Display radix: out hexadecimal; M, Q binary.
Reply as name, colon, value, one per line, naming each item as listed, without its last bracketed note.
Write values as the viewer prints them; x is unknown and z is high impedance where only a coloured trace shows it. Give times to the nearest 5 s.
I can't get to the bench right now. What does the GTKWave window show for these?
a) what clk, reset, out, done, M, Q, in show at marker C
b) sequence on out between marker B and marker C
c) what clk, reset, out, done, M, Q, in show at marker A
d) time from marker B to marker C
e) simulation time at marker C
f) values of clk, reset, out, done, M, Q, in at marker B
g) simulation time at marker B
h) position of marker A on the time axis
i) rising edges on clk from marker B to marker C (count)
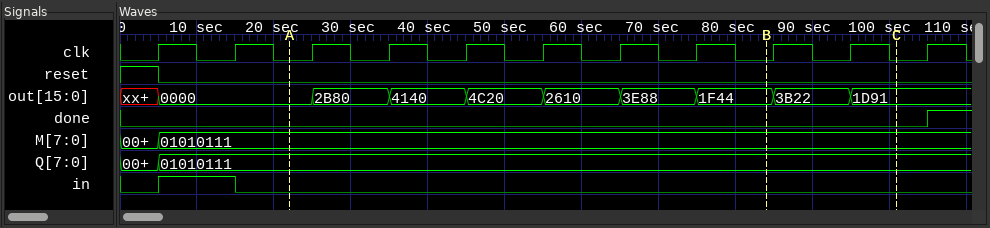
what clk, reset, out, done, M, Q, in show at marker C: clk=0, reset=0, out=1D91, done=0, M=01010111, Q=01010111, in=0
sequence on out between marker B and marker C: 1F44, 3B22, 1D91
what clk, reset, out, done, M, Q, in show at marker A: clk=0, reset=0, out=0000, done=0, M=01010111, Q=01010111, in=0
time from marker B to marker C: 15 s
simulation time at marker C: 100 s
values of clk, reset, out, done, M, Q, in at marker B: clk=0, reset=0, out=1F44, done=0, M=01010111, Q=01010111, in=0
simulation time at marker B: 85 s
position of marker A on the time axis: 20 s
rising edges on clk from marker B to marker C: 2
